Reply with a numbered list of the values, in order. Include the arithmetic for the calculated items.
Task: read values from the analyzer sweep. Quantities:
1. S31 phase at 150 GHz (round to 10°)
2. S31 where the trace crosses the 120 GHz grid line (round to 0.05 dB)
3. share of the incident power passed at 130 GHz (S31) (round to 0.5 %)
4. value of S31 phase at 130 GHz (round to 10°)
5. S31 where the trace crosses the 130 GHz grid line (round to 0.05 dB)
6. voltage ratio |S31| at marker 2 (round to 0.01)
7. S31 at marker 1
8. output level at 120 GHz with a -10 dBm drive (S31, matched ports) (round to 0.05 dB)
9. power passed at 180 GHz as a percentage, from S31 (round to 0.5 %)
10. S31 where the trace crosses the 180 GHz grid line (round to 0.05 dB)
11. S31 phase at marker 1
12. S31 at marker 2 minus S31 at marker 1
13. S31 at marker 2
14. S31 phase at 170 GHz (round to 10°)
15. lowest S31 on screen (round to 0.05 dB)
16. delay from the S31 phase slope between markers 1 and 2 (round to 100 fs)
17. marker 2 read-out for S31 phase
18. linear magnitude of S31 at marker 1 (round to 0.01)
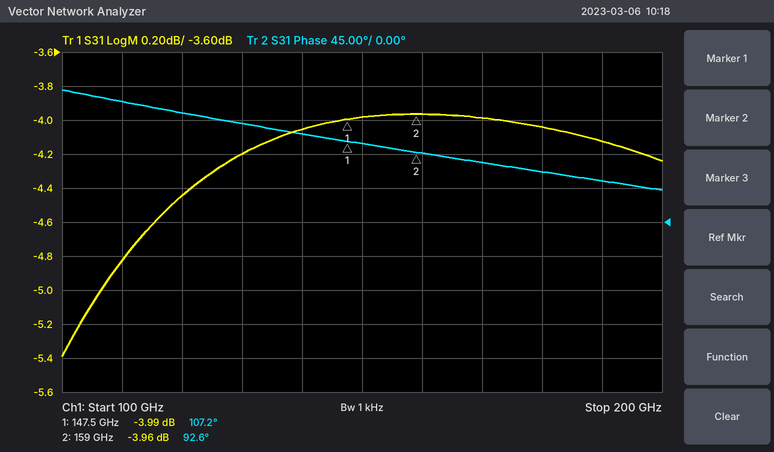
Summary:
1. 100°
2. -4.45 dB
3. 10^(-4.2/10) ≈ 38.0 %
4. 130°
5. -4.20 dB
6. 10^(-3.96/20) ≈ 0.63
7. -3.99 dB
8. -10 dBm + (-4.45 dB) = -14.45 dBm
9. 10^(-4.05/10) ≈ 39.4 %, so 39.5 % to the nearest 0.5 %
10. -4.05 dB
11. 107.2°
12. -3.96 − (-3.99) = 0.03 dB
13. -3.96 dB
14. 80°
15. -5.40 dB
16. −(92.6° − (107.2°))/(360° × 11.5 GHz) ≈ 3.5 ps
17. 92.6°
18. 10^(-3.99/20) ≈ 0.63
